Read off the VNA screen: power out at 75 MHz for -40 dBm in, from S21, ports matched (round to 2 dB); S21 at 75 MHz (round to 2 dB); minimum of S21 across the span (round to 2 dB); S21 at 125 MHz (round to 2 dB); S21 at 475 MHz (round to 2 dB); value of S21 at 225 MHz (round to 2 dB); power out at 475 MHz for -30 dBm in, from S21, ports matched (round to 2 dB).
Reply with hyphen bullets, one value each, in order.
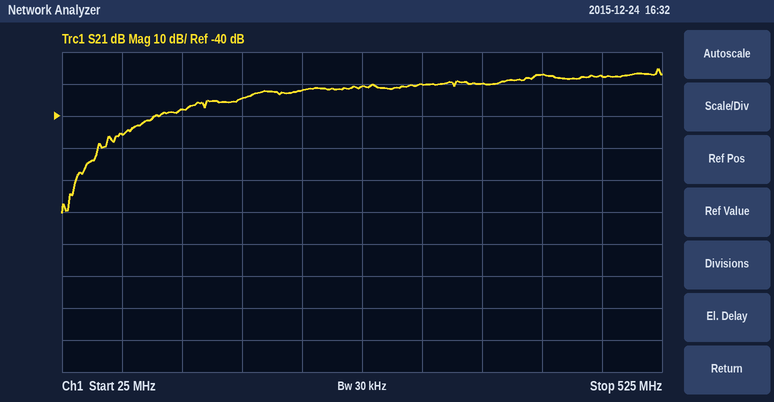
- -86 dBm
- -46 dB
- -70 dB
- -38 dB
- -28 dB
- -32 dB
- -58 dBm
